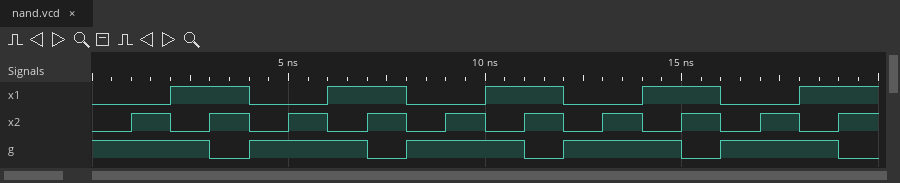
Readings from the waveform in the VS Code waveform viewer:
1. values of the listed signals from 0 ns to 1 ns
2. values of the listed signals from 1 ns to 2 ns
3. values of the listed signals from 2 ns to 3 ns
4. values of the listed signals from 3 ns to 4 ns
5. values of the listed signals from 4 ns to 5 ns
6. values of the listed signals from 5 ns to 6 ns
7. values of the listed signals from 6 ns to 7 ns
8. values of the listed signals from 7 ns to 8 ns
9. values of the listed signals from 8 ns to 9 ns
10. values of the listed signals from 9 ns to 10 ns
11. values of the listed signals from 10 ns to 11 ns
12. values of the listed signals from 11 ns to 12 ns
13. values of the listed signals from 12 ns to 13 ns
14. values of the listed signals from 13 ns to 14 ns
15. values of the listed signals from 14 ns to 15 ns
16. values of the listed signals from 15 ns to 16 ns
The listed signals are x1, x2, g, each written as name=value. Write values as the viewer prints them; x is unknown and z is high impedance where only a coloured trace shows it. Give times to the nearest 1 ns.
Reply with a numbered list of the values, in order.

1. x1=0, x2=0, g=1
2. x1=0, x2=1, g=1
3. x1=1, x2=0, g=1
4. x1=1, x2=1, g=0
5. x1=0, x2=0, g=1
6. x1=0, x2=1, g=1
7. x1=1, x2=0, g=1
8. x1=1, x2=1, g=0
9. x1=0, x2=0, g=1
10. x1=0, x2=1, g=1
11. x1=1, x2=0, g=1
12. x1=1, x2=1, g=0
13. x1=0, x2=0, g=1
14. x1=0, x2=1, g=1
15. x1=1, x2=0, g=1
16. x1=1, x2=1, g=0
